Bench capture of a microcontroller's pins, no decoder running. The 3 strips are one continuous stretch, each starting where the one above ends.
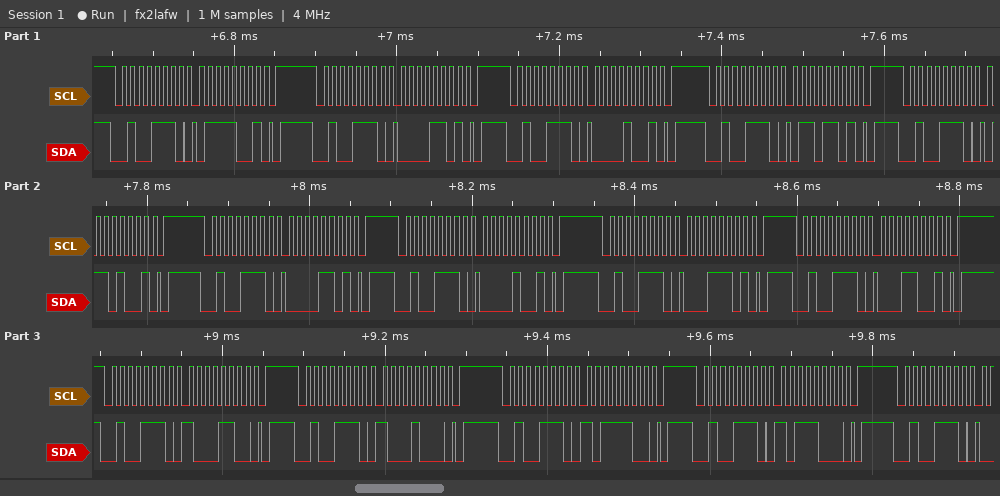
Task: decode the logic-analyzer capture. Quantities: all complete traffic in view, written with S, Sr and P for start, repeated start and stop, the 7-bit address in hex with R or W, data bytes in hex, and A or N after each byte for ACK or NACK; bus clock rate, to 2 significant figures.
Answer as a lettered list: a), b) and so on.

a) S 27W A 79 A P S 27W A 0D A P S 27W A 09 A P S 27W A 6D A P S 27W A 69 A P S 27W A 0D A P S 27W A 09 A P S 27W A 1D A P S 27W A 19 A P S 27W A 8C A P S 27W A 88 A P S 27W A BC A P S 27W A B8 A P S 27W A
b) 100 kHz
